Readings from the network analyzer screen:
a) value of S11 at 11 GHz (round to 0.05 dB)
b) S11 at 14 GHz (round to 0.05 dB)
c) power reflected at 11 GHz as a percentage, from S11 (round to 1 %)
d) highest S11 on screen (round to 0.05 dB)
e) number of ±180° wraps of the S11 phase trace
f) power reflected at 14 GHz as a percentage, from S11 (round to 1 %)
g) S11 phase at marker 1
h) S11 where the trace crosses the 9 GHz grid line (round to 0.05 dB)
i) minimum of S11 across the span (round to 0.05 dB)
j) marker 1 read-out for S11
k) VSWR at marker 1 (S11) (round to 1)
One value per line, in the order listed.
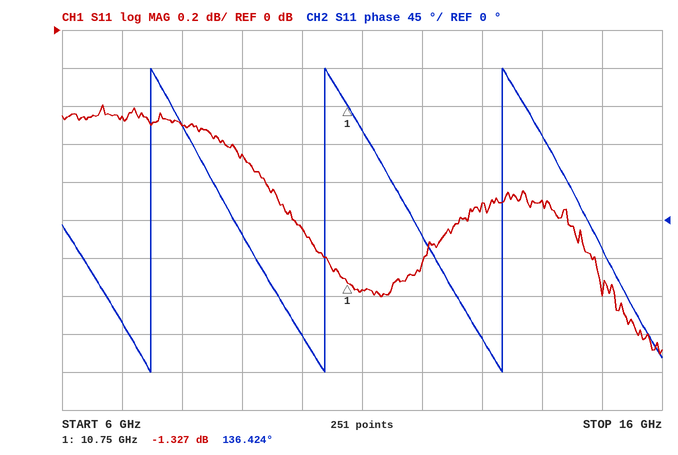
-1.35 dB
-0.90 dB
73 %
-0.40 dB
3
81 %
136.424°
-0.65 dB
-1.70 dB
-1.327 dB
13
